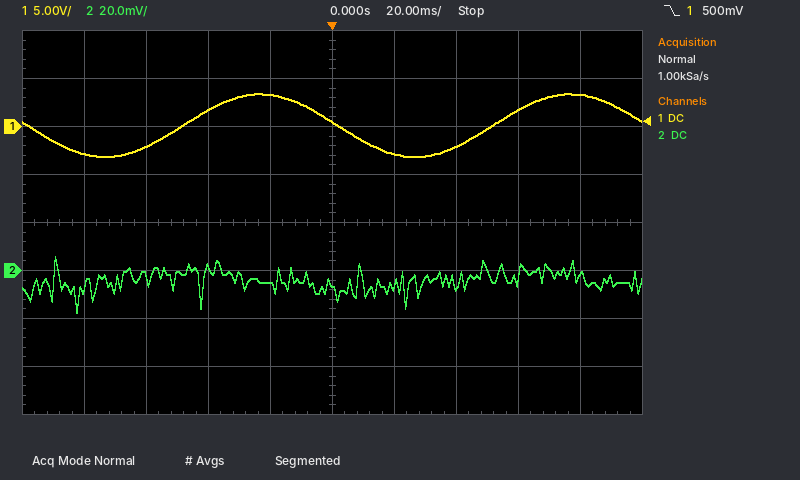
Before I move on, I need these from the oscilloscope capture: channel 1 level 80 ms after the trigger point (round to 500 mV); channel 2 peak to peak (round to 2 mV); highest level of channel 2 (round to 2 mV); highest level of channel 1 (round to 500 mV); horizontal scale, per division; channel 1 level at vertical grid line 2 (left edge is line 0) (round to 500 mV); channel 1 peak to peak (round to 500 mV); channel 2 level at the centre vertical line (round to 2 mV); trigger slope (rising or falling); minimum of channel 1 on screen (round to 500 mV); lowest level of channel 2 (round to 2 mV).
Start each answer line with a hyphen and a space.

- 3.5 V
- 24 mV
- 6 mV
- 3.5 V
- 20 ms
- -2.0 V
- 6.5 V
- -6 mV
- falling
- -3.0 V
- -18 mV
